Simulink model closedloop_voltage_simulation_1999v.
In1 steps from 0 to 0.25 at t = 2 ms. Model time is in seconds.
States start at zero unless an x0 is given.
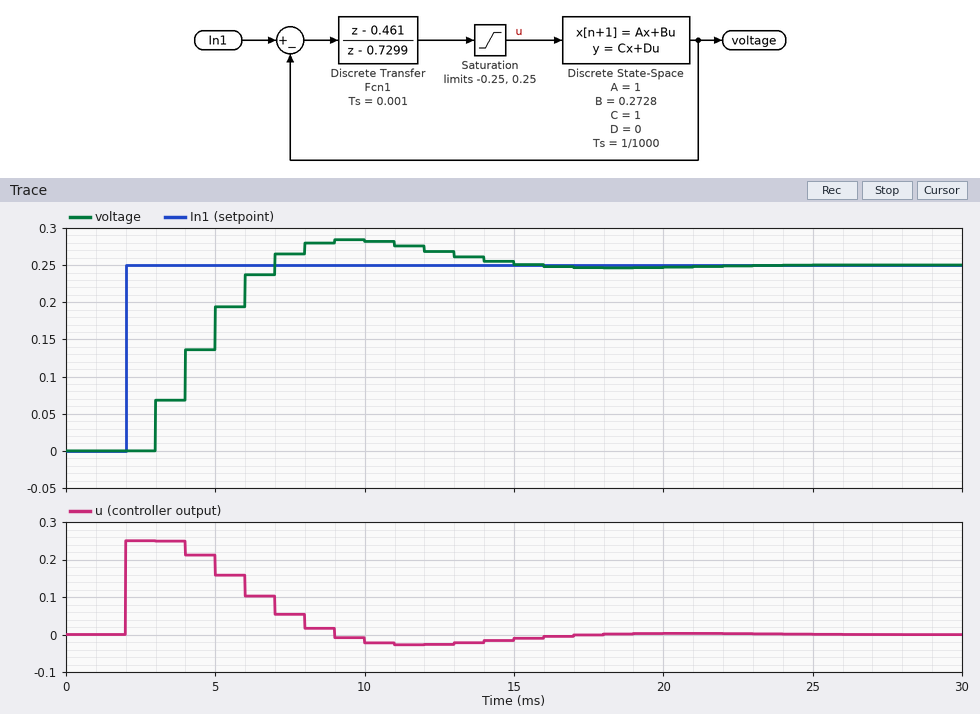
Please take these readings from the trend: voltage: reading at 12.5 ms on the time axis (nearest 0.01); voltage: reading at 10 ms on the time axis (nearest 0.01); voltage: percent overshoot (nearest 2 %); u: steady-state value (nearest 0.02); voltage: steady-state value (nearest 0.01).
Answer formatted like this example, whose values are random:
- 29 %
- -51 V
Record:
- 0.27
- 0.28
- 14 %
- 0.00
- 0.25
